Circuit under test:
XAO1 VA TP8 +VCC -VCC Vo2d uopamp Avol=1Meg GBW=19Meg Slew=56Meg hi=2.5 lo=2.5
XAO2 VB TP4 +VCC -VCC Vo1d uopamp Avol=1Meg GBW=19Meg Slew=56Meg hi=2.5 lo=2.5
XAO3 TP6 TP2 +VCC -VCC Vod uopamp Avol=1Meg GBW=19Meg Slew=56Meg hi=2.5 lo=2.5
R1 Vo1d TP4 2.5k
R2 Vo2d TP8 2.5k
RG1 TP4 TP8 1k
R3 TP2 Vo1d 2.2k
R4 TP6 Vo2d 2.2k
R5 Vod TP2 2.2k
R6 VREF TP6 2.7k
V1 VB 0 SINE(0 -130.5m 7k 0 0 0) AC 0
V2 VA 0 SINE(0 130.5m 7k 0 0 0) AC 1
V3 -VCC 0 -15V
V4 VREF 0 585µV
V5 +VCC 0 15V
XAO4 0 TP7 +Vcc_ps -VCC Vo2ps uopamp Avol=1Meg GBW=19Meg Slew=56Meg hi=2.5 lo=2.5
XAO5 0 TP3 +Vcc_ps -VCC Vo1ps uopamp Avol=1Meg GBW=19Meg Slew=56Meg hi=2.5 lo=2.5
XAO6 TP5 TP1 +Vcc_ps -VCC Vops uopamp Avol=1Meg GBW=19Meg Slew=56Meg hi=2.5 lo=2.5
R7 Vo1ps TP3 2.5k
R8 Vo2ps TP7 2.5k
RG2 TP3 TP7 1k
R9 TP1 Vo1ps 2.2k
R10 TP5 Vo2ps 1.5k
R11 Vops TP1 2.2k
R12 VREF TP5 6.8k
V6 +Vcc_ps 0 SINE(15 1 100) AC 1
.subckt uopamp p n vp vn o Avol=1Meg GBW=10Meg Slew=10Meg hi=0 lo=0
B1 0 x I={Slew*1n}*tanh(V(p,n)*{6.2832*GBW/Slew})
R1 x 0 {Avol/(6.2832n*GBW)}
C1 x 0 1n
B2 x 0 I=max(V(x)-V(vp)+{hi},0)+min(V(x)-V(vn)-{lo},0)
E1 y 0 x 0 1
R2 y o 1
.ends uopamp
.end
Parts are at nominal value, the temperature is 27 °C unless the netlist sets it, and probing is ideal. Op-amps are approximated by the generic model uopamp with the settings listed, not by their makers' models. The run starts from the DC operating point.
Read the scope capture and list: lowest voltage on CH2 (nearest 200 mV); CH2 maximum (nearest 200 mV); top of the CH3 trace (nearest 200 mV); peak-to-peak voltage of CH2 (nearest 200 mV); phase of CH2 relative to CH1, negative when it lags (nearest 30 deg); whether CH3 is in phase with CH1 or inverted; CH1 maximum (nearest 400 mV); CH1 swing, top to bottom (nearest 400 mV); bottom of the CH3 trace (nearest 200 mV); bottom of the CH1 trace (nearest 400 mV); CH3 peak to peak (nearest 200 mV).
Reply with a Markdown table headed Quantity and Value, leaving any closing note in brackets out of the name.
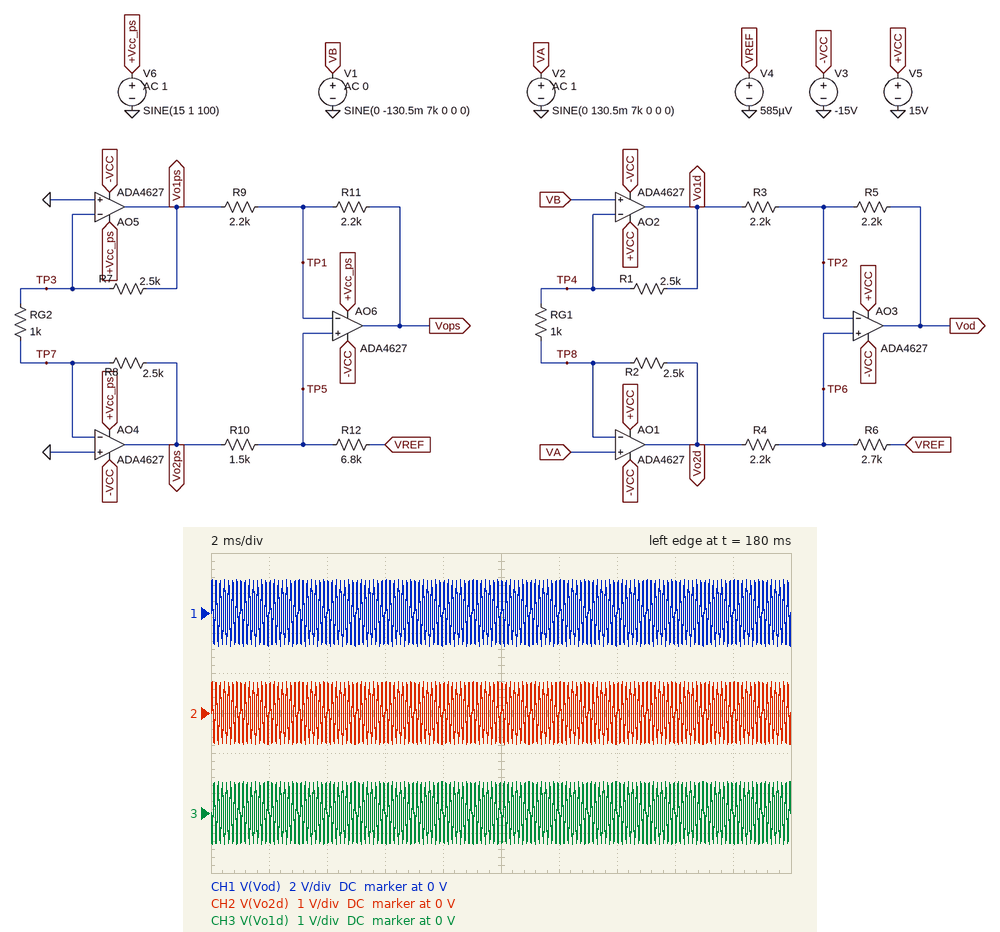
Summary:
| Quantity | Value |
|---|---|
| lowest voltage on CH2 | -800 mV |
| CH2 maximum | 800 mV |
| top of the CH3 trace | 800 mV |
| peak-to-peak voltage of CH2 | 1.6 V |
| phase of CH2 relative to CH1, negative when it lags | 0 deg |
| whether CH3 is in phase with CH1 or inverted | inverted |
| CH1 maximum | 1.6 V |
| CH1 swing, top to bottom | 3.2 V |
| bottom of the CH3 trace | -800 mV |
| bottom of the CH1 trace | -1.6 V |
| CH3 peak to peak | 1.6 V |
